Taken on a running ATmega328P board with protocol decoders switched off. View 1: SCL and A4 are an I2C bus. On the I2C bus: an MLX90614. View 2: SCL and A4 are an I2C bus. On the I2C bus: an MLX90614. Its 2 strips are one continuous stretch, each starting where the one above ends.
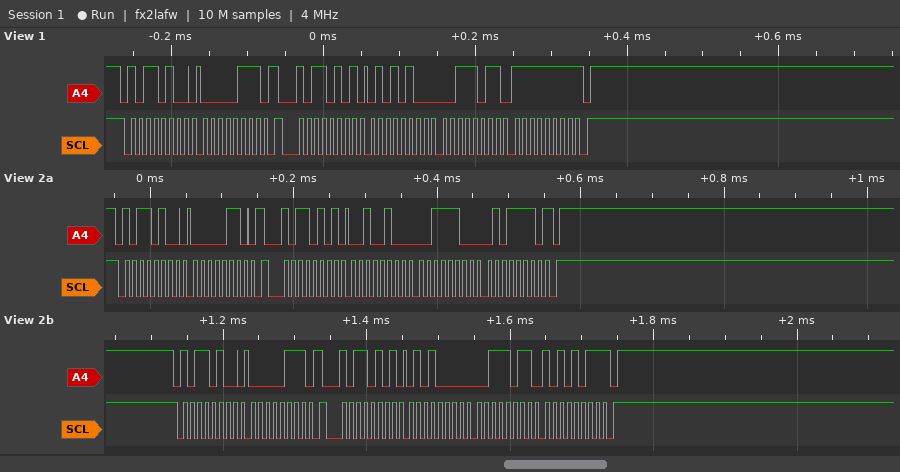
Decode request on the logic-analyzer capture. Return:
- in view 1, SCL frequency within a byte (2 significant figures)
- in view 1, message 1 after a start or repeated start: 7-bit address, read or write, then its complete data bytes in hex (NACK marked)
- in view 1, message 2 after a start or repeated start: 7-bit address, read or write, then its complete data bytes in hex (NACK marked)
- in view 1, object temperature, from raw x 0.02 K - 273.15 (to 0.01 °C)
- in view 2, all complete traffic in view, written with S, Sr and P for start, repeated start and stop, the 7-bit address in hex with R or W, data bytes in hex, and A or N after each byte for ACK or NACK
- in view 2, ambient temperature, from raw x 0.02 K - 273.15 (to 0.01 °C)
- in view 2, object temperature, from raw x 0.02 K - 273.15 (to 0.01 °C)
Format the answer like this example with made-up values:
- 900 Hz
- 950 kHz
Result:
- 100 kHz
- 0x5A write: 07
- 0x5A read: 54 3B FF NACK
- 30.61 °C
- S 5AW A 06 A Sr 5AR A 24 A 3C A 5E N P S 5AW A 07 A Sr 5AR A 50 A 3B A AB N P
- 34.77 °C
- 30.53 °C
